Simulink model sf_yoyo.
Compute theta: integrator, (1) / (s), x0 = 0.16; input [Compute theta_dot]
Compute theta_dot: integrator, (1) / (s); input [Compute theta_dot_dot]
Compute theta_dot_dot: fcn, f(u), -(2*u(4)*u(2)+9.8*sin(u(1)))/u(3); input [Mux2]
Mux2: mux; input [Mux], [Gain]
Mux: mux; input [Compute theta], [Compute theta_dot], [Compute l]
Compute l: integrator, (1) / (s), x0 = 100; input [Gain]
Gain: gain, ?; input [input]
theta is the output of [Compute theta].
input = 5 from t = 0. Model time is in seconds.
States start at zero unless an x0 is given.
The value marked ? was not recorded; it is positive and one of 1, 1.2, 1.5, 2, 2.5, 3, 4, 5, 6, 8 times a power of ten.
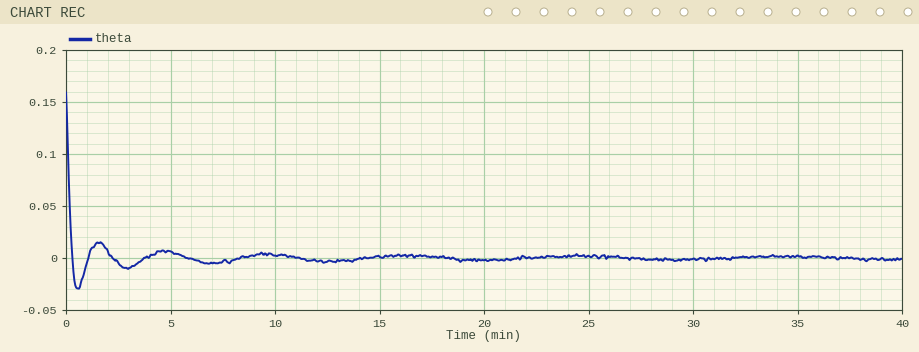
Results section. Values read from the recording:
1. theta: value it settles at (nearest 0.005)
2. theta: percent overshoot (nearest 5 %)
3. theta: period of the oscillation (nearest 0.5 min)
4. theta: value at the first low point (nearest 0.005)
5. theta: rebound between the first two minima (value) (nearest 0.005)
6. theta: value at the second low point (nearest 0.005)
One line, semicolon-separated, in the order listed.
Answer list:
0.000; 20 %; 2.5 min; -0.030; 0.015; -0.010
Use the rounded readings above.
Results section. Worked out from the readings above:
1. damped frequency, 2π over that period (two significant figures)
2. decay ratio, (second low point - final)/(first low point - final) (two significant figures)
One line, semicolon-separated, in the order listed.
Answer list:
2.5 rad/min; 0.33
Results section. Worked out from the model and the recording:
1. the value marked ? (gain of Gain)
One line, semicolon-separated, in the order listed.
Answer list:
10
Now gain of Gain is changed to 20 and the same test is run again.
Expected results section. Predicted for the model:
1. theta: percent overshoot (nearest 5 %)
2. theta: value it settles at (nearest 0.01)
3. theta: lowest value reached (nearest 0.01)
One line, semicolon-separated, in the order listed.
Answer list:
15 %; 0.00; -0.02
